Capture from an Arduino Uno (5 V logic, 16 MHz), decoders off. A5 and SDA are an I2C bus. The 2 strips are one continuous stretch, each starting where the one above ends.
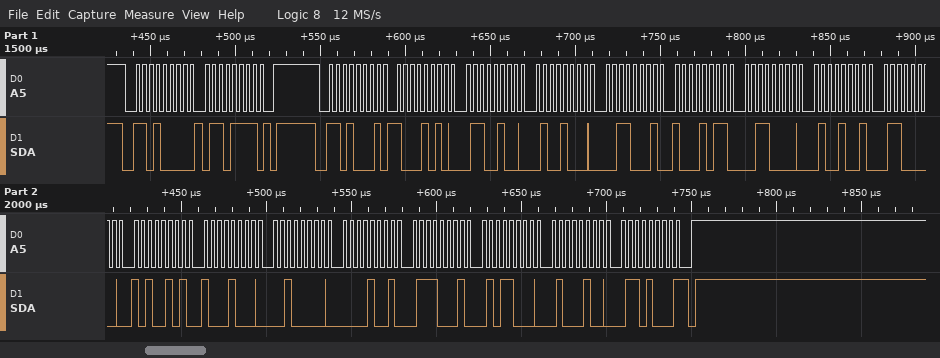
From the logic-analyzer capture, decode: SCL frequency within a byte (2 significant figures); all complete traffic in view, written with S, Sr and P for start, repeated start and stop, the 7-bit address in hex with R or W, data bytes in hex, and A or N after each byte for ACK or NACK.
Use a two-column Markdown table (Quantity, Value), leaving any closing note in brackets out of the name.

| Quantity | Value |
|---|---|
| SCL frequency within a byte | 250 kHz |
| all complete traffic in view, written with S, Sr and P for start, repeated start and stop, the 7-bit address in hex with R or W, data bytes in hex, and A or N after each byte for ACK or NACK | S 68W A 6F A P S 68R A 8A A 64 A 48 A 31 A 8B A 30 A 49 A 60 A A5 A 88 A 20 A 09 A 71 A 58 A 44 A 68 N P |
